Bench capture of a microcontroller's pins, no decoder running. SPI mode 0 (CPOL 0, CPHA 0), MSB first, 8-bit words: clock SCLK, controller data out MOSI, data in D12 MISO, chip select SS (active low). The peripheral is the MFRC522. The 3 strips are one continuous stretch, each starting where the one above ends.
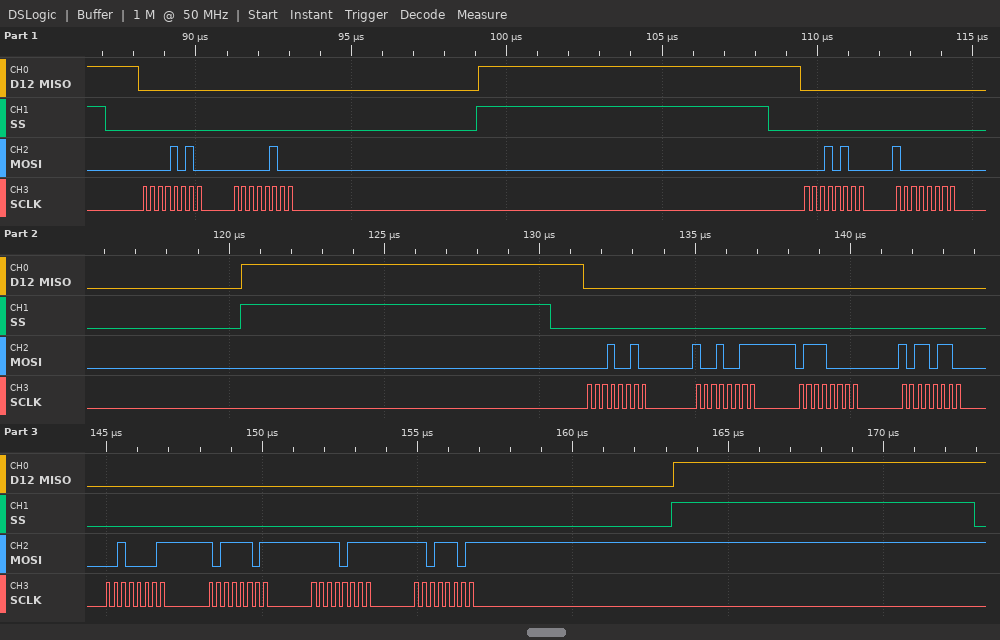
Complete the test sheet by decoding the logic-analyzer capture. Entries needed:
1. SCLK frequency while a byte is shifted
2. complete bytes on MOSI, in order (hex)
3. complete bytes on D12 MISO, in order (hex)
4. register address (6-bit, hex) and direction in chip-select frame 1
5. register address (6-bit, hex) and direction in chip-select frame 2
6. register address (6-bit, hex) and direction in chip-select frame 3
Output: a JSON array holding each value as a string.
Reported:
["4 MHz", "0A 04 14 80 12 93 70 B6 21 BD F7 DD", "00 00 00 00 00 00 00 00 00 00 00 00", "0x05 write", "0x0A write", "0x09 write"]
